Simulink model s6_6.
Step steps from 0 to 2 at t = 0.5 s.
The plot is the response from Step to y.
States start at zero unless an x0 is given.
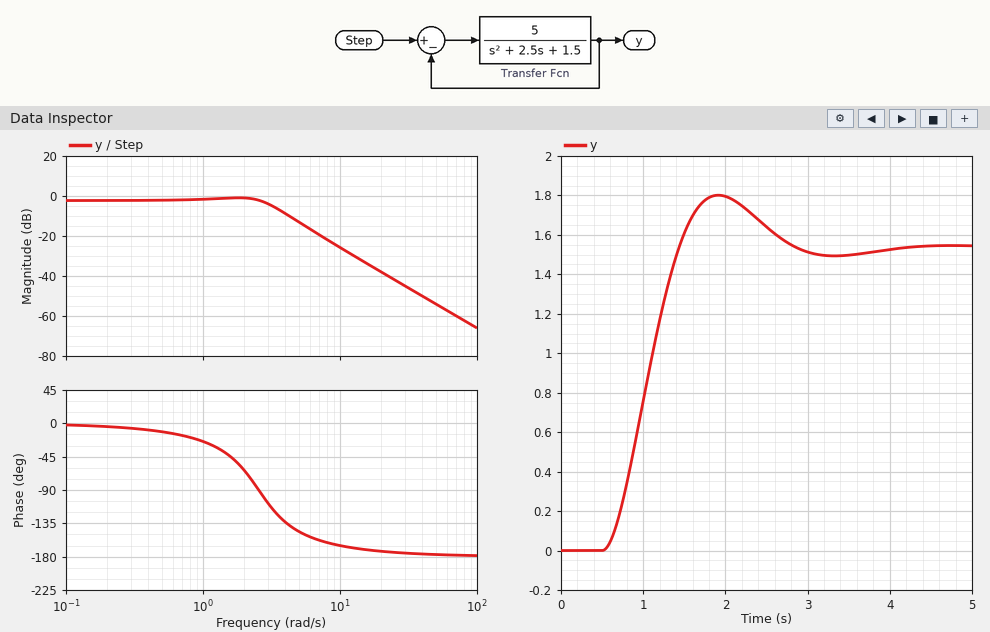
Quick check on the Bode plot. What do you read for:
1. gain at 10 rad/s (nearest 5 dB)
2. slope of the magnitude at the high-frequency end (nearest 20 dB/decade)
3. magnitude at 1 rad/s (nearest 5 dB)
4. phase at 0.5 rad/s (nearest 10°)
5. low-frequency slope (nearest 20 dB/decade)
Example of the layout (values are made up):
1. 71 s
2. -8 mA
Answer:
1. -25 dB
2. -40 dB/decade
3. 0 dB
4. -10°
5. 0 dB/decade
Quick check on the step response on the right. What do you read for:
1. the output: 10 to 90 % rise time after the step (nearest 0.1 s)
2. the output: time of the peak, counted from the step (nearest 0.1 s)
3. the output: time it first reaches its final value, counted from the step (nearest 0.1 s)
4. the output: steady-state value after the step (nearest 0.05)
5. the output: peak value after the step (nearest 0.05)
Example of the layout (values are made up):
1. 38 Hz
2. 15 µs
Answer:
1. 0.6 s
2. 1.4 s
3. 0.9 s
4. 1.55
5. 1.80
